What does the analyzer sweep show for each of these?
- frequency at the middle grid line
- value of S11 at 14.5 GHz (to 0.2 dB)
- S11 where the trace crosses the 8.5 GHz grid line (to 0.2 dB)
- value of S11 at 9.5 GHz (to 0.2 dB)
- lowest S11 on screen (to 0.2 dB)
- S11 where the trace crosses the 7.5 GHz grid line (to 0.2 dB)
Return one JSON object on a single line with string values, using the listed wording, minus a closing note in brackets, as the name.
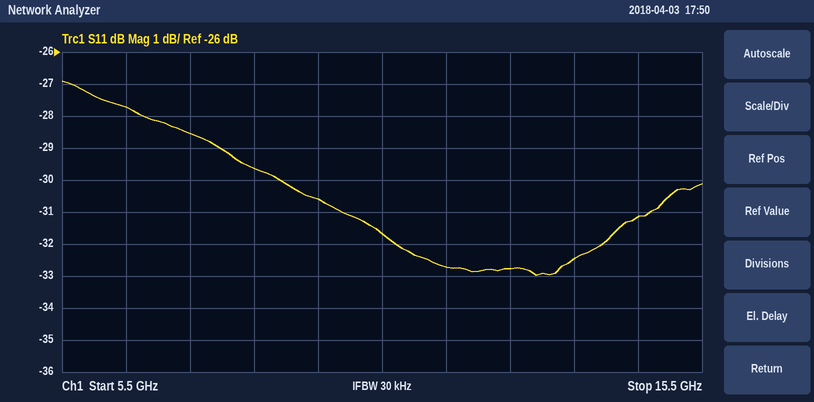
{"frequency at the middle grid line": "10.5 GHz", "value of S11 at 14.5 GHz": "-31.2 dB", "S11 where the trace crosses the 8.5 GHz grid line": "-29.6 dB", "value of S11 at 9.5 GHz": "-30.6 dB", "lowest S11 on screen": "-33.0 dB", "S11 where the trace crosses the 7.5 GHz grid line": "-28.6 dB"}
